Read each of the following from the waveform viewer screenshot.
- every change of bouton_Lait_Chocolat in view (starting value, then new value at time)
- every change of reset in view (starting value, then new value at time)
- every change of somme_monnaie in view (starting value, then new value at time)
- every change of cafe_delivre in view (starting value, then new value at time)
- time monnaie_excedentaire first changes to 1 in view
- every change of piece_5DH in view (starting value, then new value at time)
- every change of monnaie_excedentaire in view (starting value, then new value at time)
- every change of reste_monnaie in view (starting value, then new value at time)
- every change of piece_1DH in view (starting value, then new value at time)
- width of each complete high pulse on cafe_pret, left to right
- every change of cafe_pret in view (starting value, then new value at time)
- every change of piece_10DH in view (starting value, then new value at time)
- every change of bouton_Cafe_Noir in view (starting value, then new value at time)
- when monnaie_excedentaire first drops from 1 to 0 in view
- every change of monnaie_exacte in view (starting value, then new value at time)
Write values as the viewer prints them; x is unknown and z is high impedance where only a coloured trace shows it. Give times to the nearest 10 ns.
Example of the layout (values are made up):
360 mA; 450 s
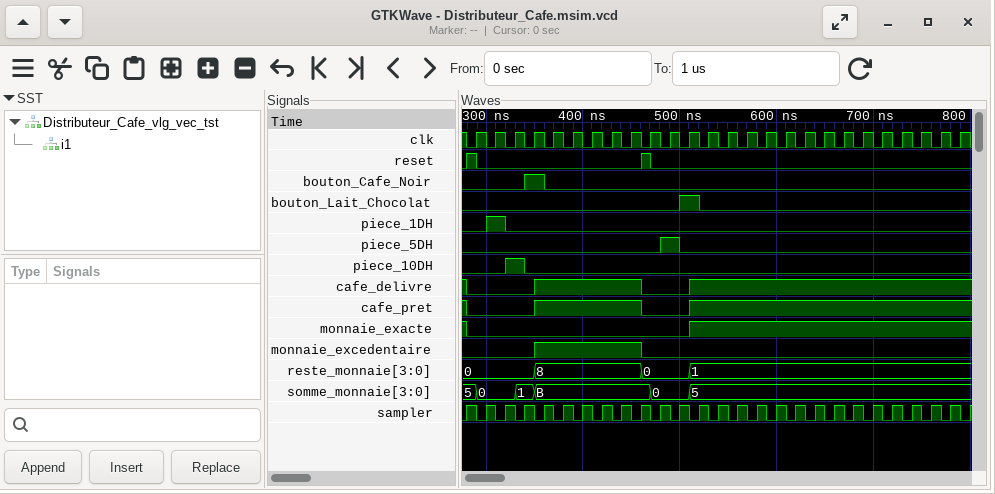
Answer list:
0, 1 at 500 ns, 0 at 520 ns; 0, 1 at 280 ns, 0 at 290 ns, 1 at 460 ns, 0 at 470 ns; 5, 0 at 290 ns, 1 at 330 ns, B at 350 ns, 0 at 470 ns, 5 at 510 ns; 1, 0 at 280 ns, 1 at 350 ns, 0 at 460 ns, 1 at 510 ns; 350 ns; 0, 1 at 480 ns, 0 at 500 ns; 0, 1 at 350 ns, 0 at 460 ns; 0, 8 at 350 ns, 0 at 460 ns, 1 at 510 ns; 0, 1 at 300 ns, 0 at 320 ns; 110 ns; 1, 0 at 280 ns, 1 at 350 ns, 0 at 460 ns, 1 at 510 ns; 0, 1 at 320 ns, 0 at 340 ns; 0, 1 at 340 ns, 0 at 360 ns; 460 ns; 1, 0 at 280 ns, 1 at 510 ns
